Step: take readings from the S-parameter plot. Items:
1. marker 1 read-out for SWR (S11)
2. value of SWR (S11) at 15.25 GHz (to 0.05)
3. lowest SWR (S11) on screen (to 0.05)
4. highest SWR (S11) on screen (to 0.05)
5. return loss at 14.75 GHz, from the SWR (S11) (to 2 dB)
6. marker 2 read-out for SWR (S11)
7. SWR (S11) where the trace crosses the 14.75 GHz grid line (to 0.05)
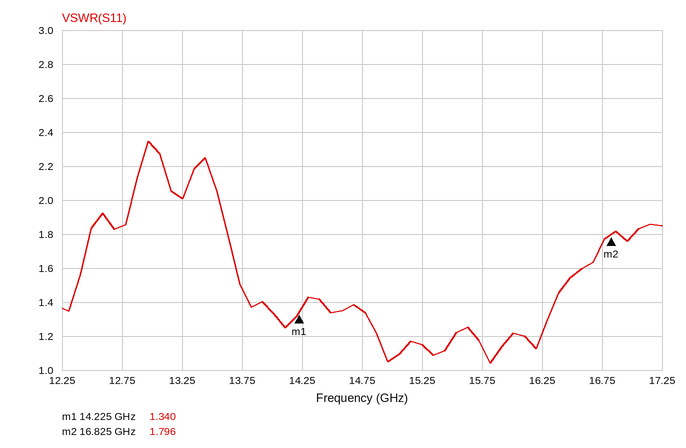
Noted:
1.340
1.15
1.05
2.35
16 dB
1.796
1.35
